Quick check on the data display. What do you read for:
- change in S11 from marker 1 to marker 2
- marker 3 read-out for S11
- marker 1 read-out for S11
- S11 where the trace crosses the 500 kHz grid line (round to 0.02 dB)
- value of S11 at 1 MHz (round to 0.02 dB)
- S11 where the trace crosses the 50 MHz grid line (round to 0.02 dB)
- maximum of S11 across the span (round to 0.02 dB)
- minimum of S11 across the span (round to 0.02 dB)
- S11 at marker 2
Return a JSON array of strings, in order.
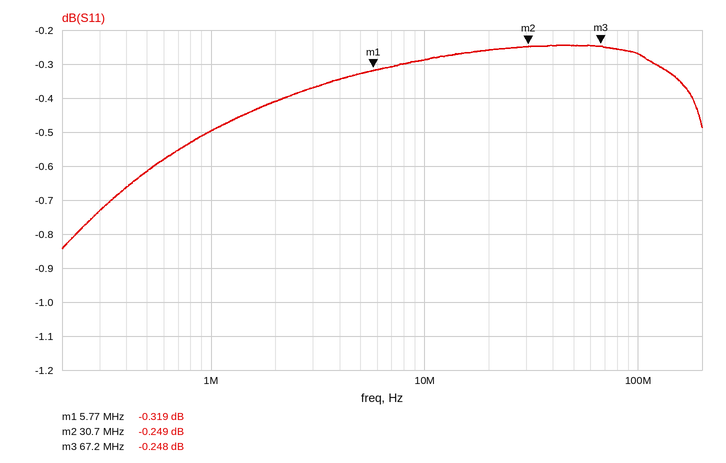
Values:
["0.070 dB", "-0.248 dB", "-0.319 dB", "-0.62 dB", "-0.50 dB", "-0.24 dB", "-0.24 dB", "-0.84 dB", "-0.249 dB"]
